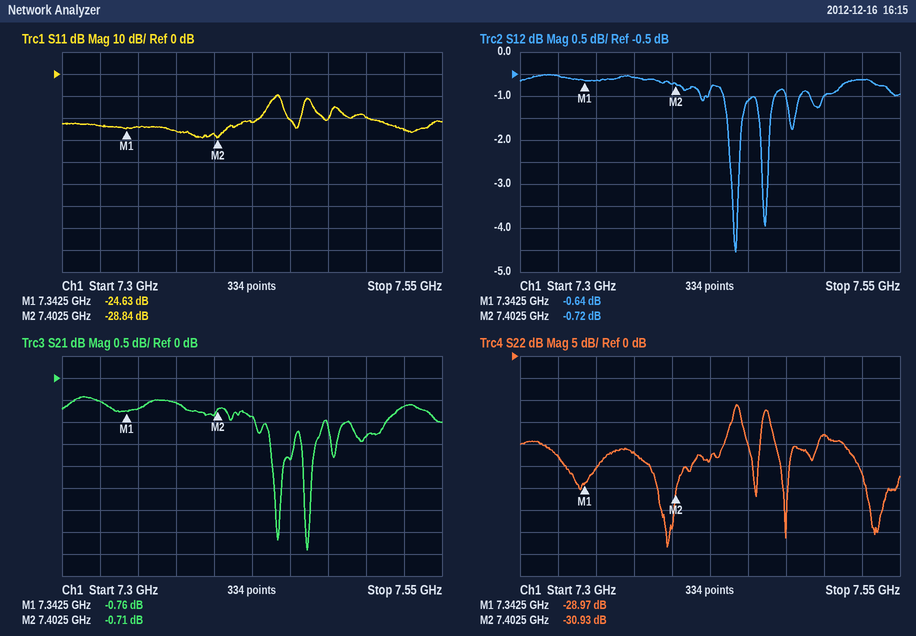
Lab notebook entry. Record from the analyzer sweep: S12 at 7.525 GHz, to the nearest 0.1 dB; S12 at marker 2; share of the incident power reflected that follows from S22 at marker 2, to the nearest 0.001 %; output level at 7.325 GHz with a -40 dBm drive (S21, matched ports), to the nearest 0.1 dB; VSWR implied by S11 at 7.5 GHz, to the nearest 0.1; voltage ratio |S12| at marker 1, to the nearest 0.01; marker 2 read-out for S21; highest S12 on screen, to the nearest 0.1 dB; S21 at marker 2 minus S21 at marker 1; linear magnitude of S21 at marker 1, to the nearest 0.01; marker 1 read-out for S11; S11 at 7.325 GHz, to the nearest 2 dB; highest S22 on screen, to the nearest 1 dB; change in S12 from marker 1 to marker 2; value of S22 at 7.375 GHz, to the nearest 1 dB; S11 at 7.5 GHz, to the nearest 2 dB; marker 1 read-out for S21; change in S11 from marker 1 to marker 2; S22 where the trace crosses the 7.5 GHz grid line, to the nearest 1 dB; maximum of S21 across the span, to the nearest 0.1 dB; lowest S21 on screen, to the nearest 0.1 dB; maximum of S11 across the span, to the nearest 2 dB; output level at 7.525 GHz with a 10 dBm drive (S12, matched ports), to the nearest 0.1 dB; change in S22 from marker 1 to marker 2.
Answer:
-0.6 dB
-0.72 dB
0.081 %
-40.5 dBm
1.2
0.93
-0.71 dB
-0.5 dB
0.05 dB
0.92
-24.63 dB
-24 dB
-11 dB
-0.08 dB
-22 dB
-20 dB
-0.76 dB
-4.21 dB
-18 dB
-0.4 dB
-3.9 dB
-10 dB
9.4 dBm
-1.96 dB
